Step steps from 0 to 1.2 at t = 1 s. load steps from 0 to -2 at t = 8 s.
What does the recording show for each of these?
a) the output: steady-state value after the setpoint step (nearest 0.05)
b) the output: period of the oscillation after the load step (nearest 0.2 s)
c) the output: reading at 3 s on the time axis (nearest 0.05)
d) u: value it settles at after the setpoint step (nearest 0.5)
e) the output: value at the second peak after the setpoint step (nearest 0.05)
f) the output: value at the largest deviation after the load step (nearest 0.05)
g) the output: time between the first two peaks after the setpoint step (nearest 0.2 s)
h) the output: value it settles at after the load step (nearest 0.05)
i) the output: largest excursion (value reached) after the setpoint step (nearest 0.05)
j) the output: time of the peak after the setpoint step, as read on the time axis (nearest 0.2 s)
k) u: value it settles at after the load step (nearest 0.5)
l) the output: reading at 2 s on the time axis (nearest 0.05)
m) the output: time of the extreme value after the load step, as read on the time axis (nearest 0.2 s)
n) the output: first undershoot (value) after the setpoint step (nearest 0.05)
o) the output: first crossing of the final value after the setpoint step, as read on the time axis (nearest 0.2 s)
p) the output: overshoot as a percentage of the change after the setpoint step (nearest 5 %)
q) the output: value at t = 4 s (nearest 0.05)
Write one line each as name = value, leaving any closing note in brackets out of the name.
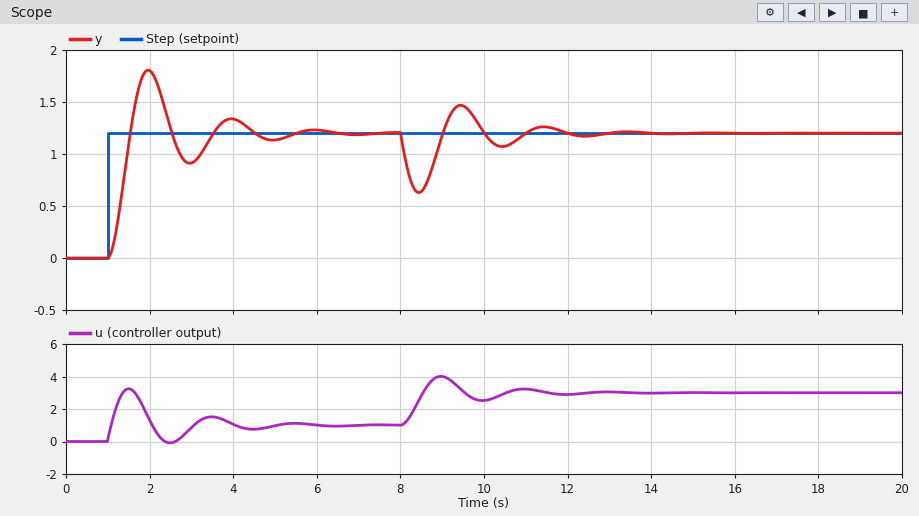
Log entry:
the output: steady-state value after the setpoint step = 1.20
the output: period of the oscillation after the load step = 2.0 s
the output: reading at 3 s on the time axis = 0.90
u: value it settles at after the setpoint step = 1.0
the output: value at the second peak after the setpoint step = 1.35
the output: value at the largest deviation after the load step = 0.65
the output: time between the first two peaks after the setpoint step = 2.0 s
the output: value it settles at after the load step = 1.20
the output: largest excursion (value reached) after the setpoint step = 1.80
the output: time of the peak after the setpoint step, as read on the time axis = 2.0 s
u: value it settles at after the load step = 3.0
the output: reading at 2 s on the time axis = 1.80
the output: time of the extreme value after the load step, as read on the time axis = 8.4 s
the output: first undershoot (value) after the setpoint step = 0.90
the output: first crossing of the final value after the setpoint step, as read on the time axis = 1.6 s
the output: overshoot as a percentage of the change after the setpoint step = 50 %
the output: value at t = 4 s = 1.35
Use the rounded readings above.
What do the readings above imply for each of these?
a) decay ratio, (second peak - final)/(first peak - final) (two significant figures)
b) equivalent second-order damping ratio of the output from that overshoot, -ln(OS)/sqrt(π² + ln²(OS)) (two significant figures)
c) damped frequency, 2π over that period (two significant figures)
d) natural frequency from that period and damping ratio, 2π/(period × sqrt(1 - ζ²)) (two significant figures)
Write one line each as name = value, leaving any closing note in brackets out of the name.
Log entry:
decay ratio, (second peak - final)/(first peak - final) = 0.25
equivalent second-order damping ratio of the output from that overshoot, -ln(OS)/sqrt(π² + ln²(OS)) = 0.22
damped frequency, 2π over that period = 3.1 rad/s
natural frequency from that period and damping ratio, 2π/(period × sqrt(1 - ζ²)) = 3.2 rad/s
